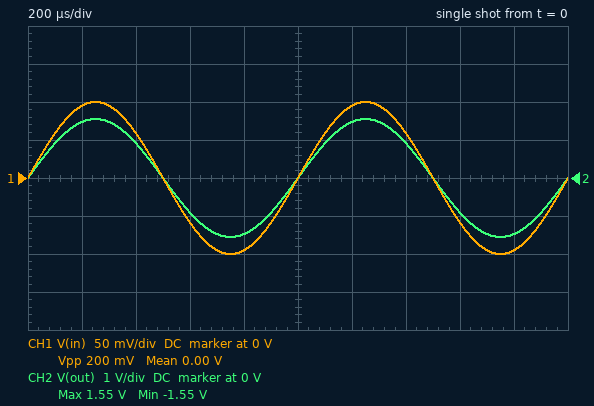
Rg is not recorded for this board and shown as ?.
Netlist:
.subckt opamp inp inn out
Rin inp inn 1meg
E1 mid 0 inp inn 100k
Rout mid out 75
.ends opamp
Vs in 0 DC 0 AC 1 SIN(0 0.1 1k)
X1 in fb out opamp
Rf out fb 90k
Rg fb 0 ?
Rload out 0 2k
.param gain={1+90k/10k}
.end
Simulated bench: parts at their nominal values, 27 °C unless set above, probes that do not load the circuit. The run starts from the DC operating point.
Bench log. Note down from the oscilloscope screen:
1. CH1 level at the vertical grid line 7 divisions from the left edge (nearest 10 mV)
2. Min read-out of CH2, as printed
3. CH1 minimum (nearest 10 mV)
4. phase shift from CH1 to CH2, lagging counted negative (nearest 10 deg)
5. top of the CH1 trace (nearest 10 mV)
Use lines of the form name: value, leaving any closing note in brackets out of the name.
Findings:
CH1 level at the vertical grid line 7 divisions from the left edge: 60 mV
Min read-out of CH2, as printed: -1.55 V
CH1 minimum: -100 mV
phase shift from CH1 to CH2, lagging counted negative: 0 deg
top of the CH1 trace: 100 mV
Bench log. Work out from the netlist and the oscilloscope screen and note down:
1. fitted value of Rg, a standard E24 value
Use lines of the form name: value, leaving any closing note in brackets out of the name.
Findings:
fitted value of Rg, a standard E24 value: 6.2 kΩ
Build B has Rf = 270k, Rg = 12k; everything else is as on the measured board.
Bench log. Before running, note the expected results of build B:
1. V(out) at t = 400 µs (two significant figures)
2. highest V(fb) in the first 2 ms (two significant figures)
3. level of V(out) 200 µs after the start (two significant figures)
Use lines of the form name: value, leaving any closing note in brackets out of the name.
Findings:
V(out) at t = 400 µs: 1.4 V
highest V(fb) in the first 2 ms: 100 mV
level of V(out) 200 µs after the start: 2.2 V
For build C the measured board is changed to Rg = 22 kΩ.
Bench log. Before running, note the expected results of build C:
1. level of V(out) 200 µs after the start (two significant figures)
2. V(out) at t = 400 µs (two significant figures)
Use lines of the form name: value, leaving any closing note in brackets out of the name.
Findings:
level of V(out) 200 µs after the start: 480 mV
V(out) at t = 400 µs: 300 mV
